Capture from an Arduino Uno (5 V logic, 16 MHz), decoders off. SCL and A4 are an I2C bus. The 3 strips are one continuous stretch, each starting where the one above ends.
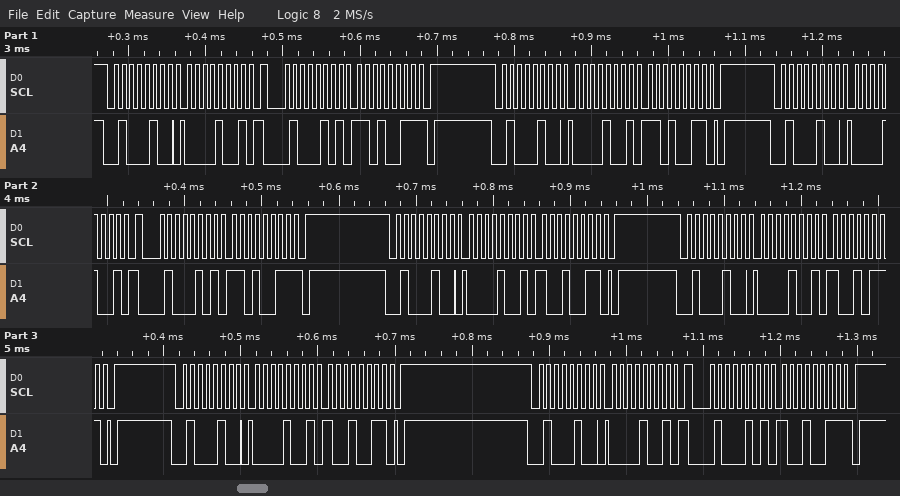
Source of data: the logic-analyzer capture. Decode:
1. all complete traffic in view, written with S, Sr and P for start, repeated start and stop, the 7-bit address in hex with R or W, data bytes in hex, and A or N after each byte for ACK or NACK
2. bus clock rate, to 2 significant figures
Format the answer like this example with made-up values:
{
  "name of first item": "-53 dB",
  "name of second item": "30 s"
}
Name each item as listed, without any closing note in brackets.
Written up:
{
  "all complete traffic in view, written with S, Sr and P for start, repeated start and stop, the 7-bit address in hex with R or W, data bytes in hex, and A or N after each byte for ACK or NACK": "S 22W A 09 A Sr 22R A D3 N P S 22W A 09 A D3 A P S 22W A 09 A Sr 22R A D3 N P S 22W A 09 A 93 A P S 22W A 09 A 97 A P S 22W A 09 A 93 A P S 22W A 09 A Sr 22R A 93 N P",
  "bus clock rate, to 2 significant figures": "100 kHz"
}
